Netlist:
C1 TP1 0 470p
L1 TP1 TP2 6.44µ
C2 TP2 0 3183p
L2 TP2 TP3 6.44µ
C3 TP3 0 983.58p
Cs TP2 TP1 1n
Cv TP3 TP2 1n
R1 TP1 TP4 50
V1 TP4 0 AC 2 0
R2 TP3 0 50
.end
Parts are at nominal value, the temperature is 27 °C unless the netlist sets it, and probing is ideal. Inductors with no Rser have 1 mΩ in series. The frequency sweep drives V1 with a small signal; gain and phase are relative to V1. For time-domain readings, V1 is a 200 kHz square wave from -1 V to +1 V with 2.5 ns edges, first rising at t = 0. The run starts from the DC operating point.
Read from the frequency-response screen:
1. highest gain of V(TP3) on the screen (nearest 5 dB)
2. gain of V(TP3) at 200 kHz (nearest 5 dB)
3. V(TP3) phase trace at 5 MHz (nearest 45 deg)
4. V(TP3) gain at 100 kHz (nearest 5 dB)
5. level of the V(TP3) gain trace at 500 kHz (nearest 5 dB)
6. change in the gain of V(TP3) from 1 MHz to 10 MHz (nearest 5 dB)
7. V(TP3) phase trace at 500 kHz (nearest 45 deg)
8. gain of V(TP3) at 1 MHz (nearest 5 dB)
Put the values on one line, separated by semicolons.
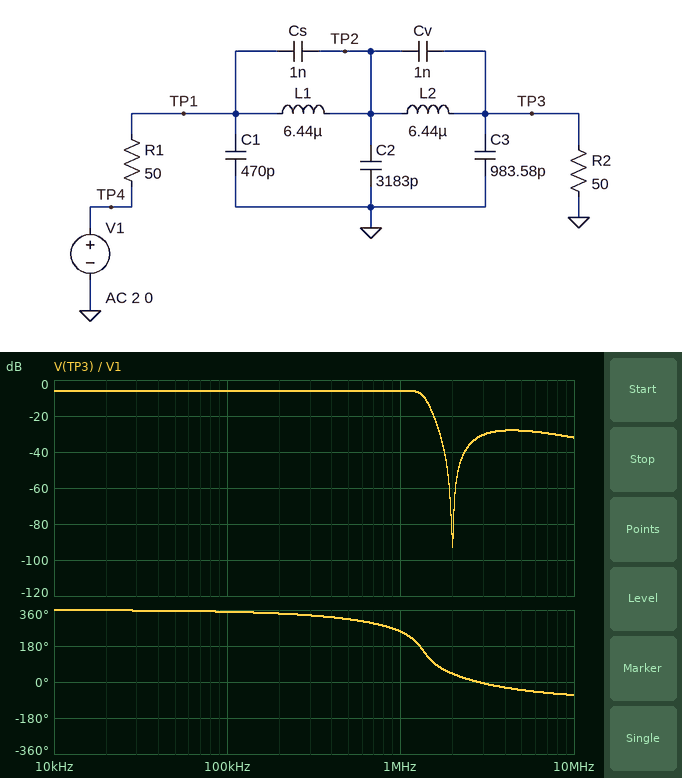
-5 dB; -5 dB; -45 deg; -5 dB; -5 dB; -25 dB; 315 deg; -5 dB
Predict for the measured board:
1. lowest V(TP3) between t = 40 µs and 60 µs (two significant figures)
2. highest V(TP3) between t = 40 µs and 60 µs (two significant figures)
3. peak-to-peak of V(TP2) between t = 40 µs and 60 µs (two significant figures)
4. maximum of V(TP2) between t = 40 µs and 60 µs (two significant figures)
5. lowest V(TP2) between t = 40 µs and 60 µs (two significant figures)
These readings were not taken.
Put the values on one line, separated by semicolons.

-670 mV; 670 mV; 1.5 V; 760 mV; -760 mV
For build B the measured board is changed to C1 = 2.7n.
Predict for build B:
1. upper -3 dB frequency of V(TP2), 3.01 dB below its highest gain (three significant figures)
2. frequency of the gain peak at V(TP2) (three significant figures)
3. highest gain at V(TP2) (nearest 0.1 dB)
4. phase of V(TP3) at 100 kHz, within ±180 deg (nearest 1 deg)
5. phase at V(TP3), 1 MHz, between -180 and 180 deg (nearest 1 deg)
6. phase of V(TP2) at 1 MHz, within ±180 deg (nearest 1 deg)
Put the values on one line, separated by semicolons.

1.41 MHz; 1.30 MHz; -1.0 dB; -11 deg; -129 deg; -70 deg
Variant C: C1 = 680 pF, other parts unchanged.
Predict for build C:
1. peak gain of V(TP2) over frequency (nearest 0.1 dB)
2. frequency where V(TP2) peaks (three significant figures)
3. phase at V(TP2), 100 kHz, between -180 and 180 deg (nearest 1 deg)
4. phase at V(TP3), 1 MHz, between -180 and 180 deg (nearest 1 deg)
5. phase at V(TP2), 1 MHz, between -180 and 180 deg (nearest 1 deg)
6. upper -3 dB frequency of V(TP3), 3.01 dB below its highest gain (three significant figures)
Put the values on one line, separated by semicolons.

-1.8 dB; 1.27 MHz; -4 deg; -110 deg; -52 deg; 1.36 MHz
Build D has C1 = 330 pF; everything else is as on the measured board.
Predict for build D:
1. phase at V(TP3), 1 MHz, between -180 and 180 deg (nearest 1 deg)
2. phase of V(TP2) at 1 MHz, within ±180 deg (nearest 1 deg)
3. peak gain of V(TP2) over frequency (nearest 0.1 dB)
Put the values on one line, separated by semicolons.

-107 deg; -48 deg; -2.1 dB
